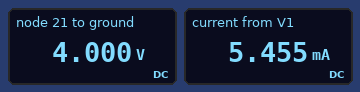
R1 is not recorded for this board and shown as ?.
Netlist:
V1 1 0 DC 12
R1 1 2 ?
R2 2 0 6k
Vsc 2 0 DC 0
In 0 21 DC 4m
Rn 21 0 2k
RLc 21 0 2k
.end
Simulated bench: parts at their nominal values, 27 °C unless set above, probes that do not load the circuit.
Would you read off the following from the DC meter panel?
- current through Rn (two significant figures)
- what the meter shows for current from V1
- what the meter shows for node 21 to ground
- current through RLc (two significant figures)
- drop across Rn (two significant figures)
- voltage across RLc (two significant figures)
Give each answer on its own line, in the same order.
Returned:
2.0 mA
5.455 mA
4.000 V
2.0 mA
4.0 V
4.0 V
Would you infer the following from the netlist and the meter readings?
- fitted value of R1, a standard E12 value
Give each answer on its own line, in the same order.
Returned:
2.2 kΩ
